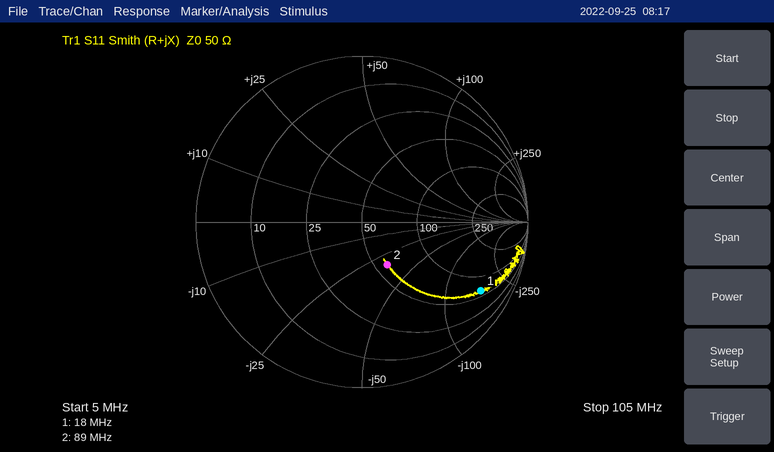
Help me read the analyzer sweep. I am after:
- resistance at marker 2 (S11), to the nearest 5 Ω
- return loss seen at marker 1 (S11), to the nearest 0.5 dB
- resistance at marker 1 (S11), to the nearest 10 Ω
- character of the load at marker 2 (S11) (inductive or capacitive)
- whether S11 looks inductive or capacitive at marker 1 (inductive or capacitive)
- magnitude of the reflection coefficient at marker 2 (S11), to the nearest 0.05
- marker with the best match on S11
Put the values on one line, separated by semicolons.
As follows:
60 Ω; 1.5 dB; 60 Ω; capacitive; capacitive; 0.30; marker 2
